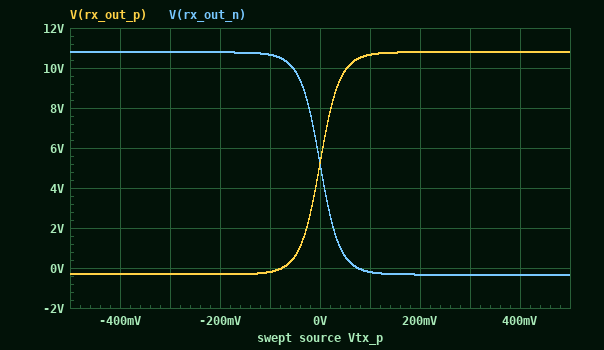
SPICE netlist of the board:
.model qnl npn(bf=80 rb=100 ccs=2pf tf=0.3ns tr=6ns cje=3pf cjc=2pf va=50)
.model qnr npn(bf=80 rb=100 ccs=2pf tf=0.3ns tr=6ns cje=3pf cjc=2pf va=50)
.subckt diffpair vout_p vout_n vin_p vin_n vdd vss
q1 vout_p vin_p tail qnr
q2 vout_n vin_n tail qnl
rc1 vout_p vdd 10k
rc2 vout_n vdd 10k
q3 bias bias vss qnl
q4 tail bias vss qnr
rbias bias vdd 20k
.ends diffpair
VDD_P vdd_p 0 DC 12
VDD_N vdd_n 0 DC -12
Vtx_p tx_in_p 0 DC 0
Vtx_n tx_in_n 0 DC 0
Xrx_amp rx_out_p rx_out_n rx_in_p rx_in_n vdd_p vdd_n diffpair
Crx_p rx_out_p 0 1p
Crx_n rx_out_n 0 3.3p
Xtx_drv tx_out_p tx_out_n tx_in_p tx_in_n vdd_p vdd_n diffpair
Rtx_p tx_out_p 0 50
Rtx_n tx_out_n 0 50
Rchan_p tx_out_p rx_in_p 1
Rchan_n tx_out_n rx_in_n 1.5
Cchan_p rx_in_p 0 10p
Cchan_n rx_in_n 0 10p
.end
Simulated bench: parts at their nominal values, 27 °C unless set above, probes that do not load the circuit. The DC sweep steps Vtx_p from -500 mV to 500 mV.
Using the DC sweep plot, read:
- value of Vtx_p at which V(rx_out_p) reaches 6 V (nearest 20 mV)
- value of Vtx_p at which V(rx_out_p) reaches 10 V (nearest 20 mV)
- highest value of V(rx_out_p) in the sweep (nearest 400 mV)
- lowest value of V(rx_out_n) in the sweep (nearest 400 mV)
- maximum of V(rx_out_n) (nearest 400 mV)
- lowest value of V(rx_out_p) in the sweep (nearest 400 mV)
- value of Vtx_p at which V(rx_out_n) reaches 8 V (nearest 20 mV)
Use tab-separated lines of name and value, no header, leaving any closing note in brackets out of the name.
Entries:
value of Vtx_p at which V(rx_out_p) reaches 6 V	0 V
value of Vtx_p at which V(rx_out_p) reaches 10 V	60 mV
highest value of V(rx_out_p) in the sweep	10.8 V
lowest value of V(rx_out_n) in the sweep	-400 mV
maximum of V(rx_out_n)	10.8 V
lowest value of V(rx_out_p) in the sweep	-400 mV
value of Vtx_p at which V(rx_out_n) reaches 8 V	-20 mV
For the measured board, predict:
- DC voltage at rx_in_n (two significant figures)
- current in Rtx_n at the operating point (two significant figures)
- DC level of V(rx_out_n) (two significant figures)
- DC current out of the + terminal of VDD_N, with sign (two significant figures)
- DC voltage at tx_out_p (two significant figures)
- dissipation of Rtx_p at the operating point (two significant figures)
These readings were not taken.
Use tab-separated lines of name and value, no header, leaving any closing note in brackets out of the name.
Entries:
DC voltage at rx_in_n	26 mV
current in Rtx_n at the operating point	510 µA
DC level of V(rx_out_n)	5.2 V
DC current out of the + terminal of VDD_N, with sign	-5.1 mA
DC voltage at tx_out_p	26 mV
dissipation of Rtx_p at the operating point	13 µW
